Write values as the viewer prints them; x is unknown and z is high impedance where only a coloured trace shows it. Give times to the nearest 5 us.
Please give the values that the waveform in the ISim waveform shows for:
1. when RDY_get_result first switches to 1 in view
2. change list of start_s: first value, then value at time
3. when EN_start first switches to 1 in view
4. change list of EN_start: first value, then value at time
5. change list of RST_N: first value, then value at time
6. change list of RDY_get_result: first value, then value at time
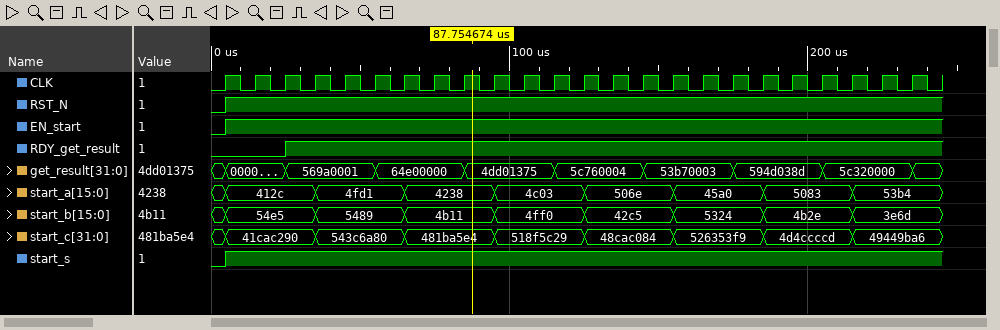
25 us
0, 1 at 5 us
5 us
0, 1 at 5 us
0, 1 at 5 us
0, 1 at 25 us
